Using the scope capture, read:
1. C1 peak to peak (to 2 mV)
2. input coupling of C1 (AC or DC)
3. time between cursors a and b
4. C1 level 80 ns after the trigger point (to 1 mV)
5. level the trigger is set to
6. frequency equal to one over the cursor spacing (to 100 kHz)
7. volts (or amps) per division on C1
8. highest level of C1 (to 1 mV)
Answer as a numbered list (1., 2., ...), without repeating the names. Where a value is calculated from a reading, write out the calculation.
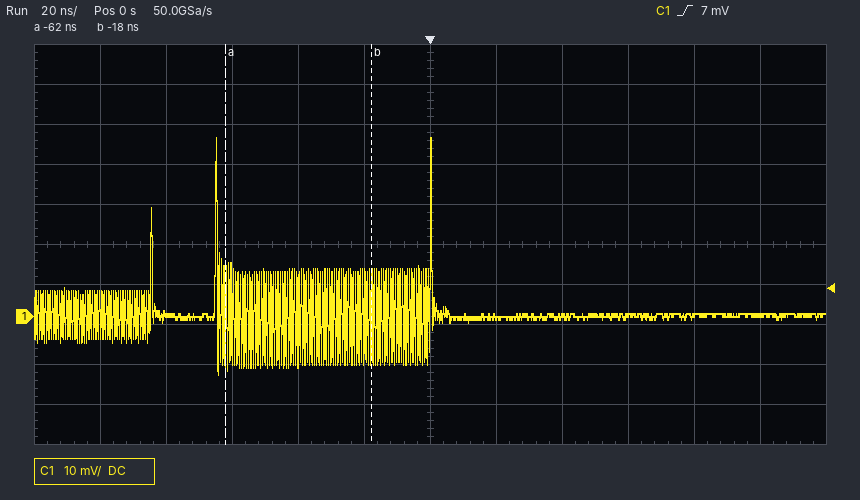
1. 60 mV
2. DC
3. -18 ns − (-62 ns) = 44 ns
4. 0 mV
5. 7 mV
6. 1 / 44 ns ≈ 22.7 MHz
7. 10 mV
8. 45 mV
